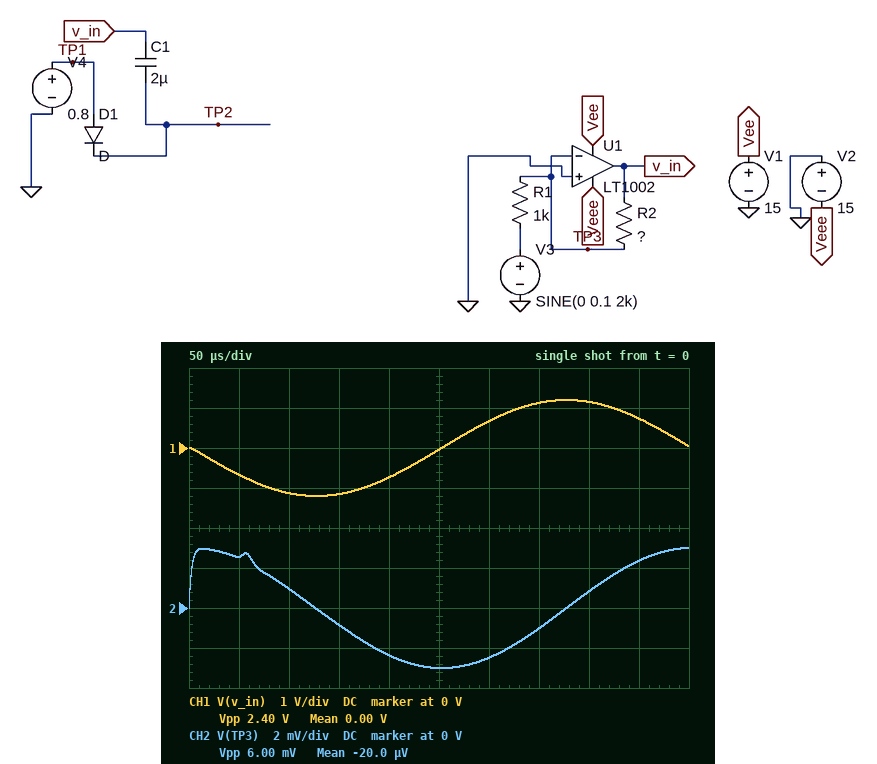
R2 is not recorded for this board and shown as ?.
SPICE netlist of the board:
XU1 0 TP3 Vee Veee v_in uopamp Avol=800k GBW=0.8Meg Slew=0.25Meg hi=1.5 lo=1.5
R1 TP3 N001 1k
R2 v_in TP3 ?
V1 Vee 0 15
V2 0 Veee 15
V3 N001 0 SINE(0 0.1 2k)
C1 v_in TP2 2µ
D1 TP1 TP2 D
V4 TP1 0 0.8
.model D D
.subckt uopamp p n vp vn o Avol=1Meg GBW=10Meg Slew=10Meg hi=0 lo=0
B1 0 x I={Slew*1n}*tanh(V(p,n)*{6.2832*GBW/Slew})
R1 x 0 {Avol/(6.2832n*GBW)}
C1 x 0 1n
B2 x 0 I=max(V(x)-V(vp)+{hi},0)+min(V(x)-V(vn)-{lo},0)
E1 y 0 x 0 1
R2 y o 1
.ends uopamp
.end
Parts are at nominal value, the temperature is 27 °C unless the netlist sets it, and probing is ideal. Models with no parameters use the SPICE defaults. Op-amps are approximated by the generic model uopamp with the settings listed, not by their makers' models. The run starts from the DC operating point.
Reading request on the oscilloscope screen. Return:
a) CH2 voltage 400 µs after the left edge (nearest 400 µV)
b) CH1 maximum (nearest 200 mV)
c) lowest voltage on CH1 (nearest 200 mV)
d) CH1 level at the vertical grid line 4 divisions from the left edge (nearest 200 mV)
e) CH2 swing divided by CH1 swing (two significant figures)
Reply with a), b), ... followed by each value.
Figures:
a) 800 µV
b) 1.2 V
c) -1.2 V
d) -800 mV
e) 0.0025
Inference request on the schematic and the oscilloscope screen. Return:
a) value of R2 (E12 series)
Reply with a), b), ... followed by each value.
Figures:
a) 12 kΩ
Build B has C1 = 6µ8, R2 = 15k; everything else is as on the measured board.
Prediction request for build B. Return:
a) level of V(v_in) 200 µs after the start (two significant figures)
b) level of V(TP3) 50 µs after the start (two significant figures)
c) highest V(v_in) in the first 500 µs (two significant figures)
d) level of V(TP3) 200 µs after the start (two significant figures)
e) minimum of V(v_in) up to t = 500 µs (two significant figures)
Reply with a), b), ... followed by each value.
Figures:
a) -930 mV
b) 4.9 mV
c) 1.5 V
d) -2.9 mV
e) -1.5 V
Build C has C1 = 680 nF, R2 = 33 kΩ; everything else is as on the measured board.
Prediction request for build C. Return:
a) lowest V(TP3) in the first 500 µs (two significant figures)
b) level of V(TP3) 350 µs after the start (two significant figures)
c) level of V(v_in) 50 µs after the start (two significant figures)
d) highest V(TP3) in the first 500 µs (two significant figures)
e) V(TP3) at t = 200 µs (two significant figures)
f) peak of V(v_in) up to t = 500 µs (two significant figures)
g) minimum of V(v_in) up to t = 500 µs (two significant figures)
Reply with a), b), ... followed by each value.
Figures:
a) -8.3 mV
b) -3.2 mV
c) -1.7 V
d) 8.4 mV
e) -6.2 mV
f) 3.3 V
g) -3.3 V
